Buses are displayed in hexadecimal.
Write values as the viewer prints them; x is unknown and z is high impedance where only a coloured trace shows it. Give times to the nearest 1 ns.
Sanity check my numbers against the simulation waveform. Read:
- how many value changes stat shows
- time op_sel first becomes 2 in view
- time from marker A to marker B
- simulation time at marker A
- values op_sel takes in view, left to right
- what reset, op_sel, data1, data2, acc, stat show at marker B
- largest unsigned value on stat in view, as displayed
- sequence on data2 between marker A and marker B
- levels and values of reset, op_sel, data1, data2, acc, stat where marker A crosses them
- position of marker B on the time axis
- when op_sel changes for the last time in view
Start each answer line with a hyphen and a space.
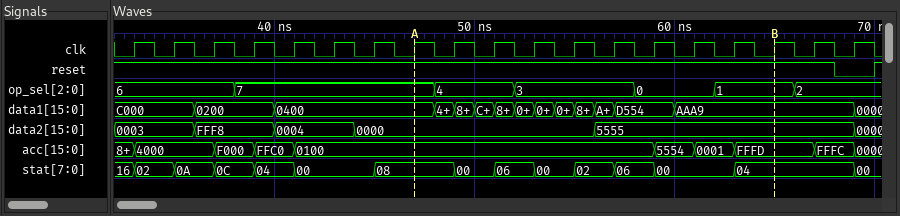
- 14
- 66 ns
- 18 ns
- 47 ns
- 6, 7, 4, 3, 0, 1, 2
- reset=1, op_sel=1, data1=AAA9, data2=5555, acc=FFFD, stat=04
- 16
- 0000, 5555
- reset=1, op_sel=7, data1=0400, data2=0000, acc=0100, stat=08
- 65 ns
- 66 ns
